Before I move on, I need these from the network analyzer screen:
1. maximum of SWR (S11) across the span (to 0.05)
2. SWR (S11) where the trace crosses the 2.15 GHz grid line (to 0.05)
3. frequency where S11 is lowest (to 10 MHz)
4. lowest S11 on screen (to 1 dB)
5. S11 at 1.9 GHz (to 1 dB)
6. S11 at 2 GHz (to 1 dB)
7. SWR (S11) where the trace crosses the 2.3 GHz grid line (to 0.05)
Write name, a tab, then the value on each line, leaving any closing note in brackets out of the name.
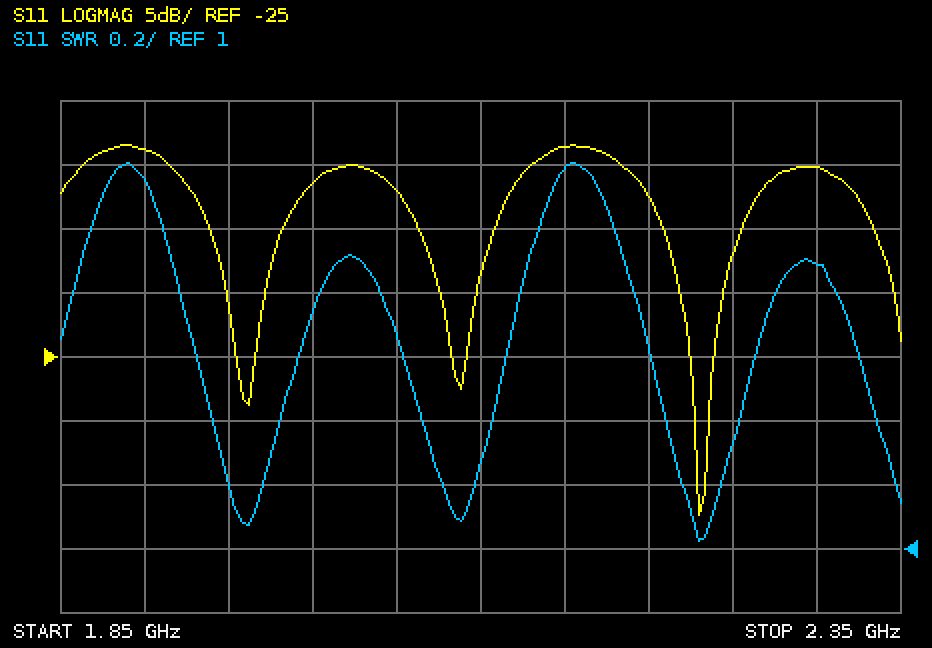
maximum of SWR (S11) across the span	2.20
SWR (S11) where the trace crosses the 2.15 GHz grid line	2.20
frequency where S11 is lowest	2.23 GHz
lowest S11 on screen	-37 dB
S11 at 1.9 GHz	-9 dB
S11 at 2 GHz	-11 dB
SWR (S11) where the trace crosses the 2.3 GHz grid line	1.90
